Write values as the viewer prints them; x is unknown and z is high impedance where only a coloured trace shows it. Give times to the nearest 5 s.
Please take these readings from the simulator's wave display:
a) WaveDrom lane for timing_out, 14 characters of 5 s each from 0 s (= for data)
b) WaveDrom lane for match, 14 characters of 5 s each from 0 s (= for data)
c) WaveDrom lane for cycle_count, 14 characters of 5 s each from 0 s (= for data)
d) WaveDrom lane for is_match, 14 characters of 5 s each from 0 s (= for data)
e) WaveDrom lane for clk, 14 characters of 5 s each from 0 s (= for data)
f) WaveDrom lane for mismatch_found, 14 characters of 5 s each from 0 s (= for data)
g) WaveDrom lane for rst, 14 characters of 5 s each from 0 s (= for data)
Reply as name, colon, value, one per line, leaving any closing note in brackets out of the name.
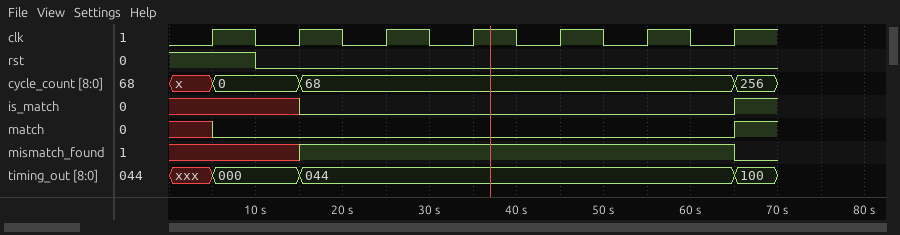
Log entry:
WaveDrom lane for timing_out, 14 characters of 5 s each from 0 s: {name: 'timing_out', wave: 'x=.=.........=', data: '000 044 100'}
WaveDrom lane for match, 14 characters of 5 s each from 0 s: {name: 'match', wave: 'x0...........1'}
WaveDrom lane for cycle_count, 14 characters of 5 s each from 0 s: {name: 'cycle_count', wave: 'x=.=.........=', data: '0 68 256'}
WaveDrom lane for is_match, 14 characters of 5 s each from 0 s: {name: 'is_match', wave: 'x..0.........1'}
WaveDrom lane for clk, 14 characters of 5 s each from 0 s: {name: 'clk', wave: '01010101010101'}
WaveDrom lane for mismatch_found, 14 characters of 5 s each from 0 s: {name: 'mismatch_found', wave: 'x..1.........0'}
WaveDrom lane for rst, 14 characters of 5 s each from 0 s: {name: 'rst', wave: '1.0...........'}
